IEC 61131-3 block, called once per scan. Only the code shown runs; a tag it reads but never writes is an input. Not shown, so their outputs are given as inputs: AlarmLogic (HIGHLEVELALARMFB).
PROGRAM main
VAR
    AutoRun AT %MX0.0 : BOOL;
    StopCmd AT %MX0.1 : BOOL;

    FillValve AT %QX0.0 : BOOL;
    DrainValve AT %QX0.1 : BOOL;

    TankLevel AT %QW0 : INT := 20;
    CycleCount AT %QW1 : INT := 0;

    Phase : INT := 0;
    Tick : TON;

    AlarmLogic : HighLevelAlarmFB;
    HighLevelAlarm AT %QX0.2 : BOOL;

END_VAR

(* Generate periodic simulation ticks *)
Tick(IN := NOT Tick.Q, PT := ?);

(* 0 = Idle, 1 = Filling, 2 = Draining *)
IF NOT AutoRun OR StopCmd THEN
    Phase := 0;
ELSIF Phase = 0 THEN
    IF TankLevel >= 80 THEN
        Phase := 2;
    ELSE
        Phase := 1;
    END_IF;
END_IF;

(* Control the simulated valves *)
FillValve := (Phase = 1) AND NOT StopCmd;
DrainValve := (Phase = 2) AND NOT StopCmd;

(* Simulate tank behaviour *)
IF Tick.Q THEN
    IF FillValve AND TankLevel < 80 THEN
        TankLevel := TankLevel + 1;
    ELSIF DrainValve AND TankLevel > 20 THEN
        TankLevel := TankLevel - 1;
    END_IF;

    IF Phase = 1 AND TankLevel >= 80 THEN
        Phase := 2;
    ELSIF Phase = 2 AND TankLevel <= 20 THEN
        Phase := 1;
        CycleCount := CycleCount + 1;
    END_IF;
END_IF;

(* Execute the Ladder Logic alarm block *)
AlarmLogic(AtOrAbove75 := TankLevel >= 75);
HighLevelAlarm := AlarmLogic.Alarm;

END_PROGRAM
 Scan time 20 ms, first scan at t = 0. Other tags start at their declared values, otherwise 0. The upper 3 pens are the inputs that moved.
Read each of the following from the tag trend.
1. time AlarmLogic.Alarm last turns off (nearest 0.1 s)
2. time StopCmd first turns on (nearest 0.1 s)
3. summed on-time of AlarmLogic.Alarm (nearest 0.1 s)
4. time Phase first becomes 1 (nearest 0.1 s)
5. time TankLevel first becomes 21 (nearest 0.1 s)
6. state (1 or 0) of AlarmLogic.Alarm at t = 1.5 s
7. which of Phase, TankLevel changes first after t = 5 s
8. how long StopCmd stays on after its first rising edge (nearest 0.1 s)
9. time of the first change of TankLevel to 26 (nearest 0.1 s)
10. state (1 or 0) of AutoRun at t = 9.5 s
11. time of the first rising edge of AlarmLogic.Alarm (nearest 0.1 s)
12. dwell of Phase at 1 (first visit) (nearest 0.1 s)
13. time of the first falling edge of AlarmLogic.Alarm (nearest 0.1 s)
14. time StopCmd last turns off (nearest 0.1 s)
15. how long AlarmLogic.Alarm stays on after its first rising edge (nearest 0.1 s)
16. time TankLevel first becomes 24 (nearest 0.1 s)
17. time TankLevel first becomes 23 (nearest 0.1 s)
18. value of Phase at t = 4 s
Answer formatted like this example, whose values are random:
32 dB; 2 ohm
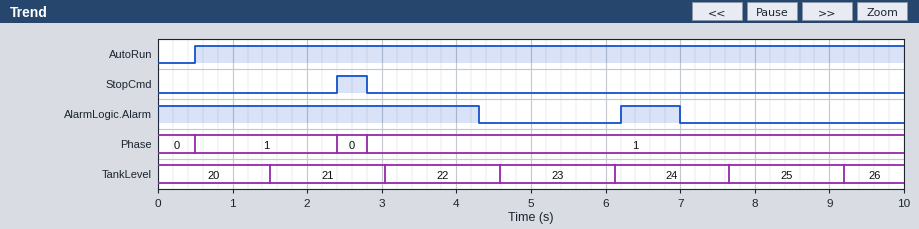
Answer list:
7.0 s; 2.4 s; 5.1 s; 0.5 s; 1.5 s; 1; TankLevel; 0.4 s; 9.2 s; 1; 6.2 s; 1.9 s; 4.3 s; 2.8 s; 0.8 s; 6.1 s; 4.6 s; 1
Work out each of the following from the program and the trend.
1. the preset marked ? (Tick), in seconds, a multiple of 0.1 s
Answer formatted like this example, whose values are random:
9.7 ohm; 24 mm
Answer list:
1.5 s
